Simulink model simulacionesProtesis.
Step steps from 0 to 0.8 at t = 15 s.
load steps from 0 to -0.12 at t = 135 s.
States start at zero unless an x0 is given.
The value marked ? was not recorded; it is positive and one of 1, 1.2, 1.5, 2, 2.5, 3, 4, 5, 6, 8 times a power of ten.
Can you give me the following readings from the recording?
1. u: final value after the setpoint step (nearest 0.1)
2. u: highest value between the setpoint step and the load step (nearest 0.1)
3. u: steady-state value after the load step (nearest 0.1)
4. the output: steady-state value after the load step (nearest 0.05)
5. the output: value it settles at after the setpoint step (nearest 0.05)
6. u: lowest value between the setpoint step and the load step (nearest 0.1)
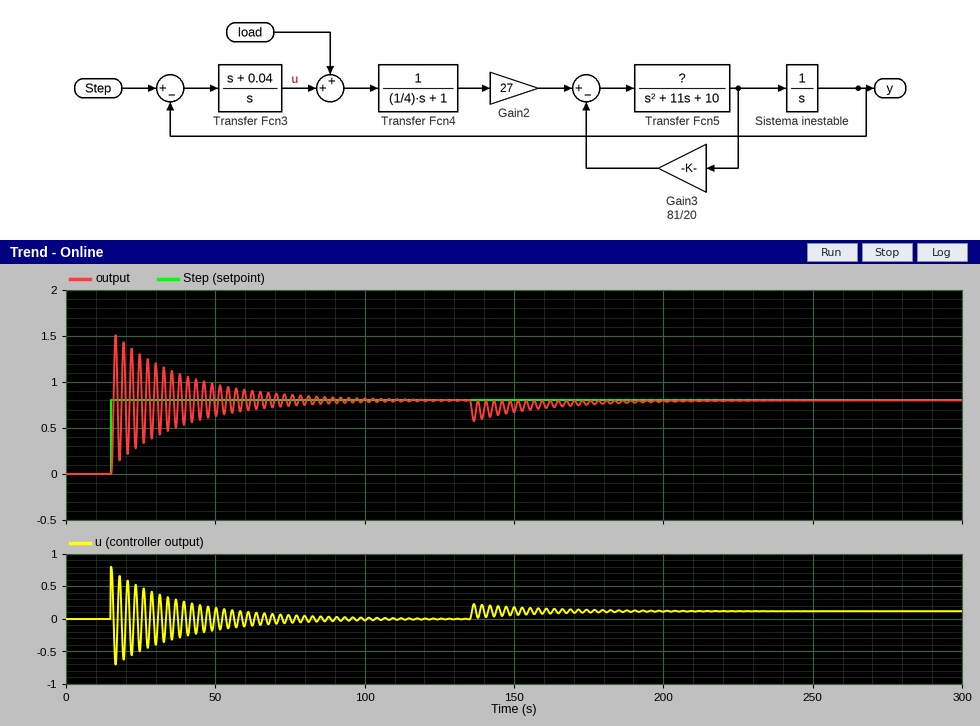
0.0
0.8
0.1
0.80
0.80
-0.7
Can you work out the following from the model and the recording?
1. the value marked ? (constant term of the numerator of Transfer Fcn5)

3
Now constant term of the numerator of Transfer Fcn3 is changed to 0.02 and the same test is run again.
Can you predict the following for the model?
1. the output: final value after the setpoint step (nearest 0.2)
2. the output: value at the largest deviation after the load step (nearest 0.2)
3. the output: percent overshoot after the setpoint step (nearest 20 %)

0.8
0.6
80 %
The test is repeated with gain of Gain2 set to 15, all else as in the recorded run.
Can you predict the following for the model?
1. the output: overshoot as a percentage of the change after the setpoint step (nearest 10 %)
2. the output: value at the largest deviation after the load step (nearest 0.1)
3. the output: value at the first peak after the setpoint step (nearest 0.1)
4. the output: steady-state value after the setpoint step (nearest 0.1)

50 %
0.6
1.2
0.8
